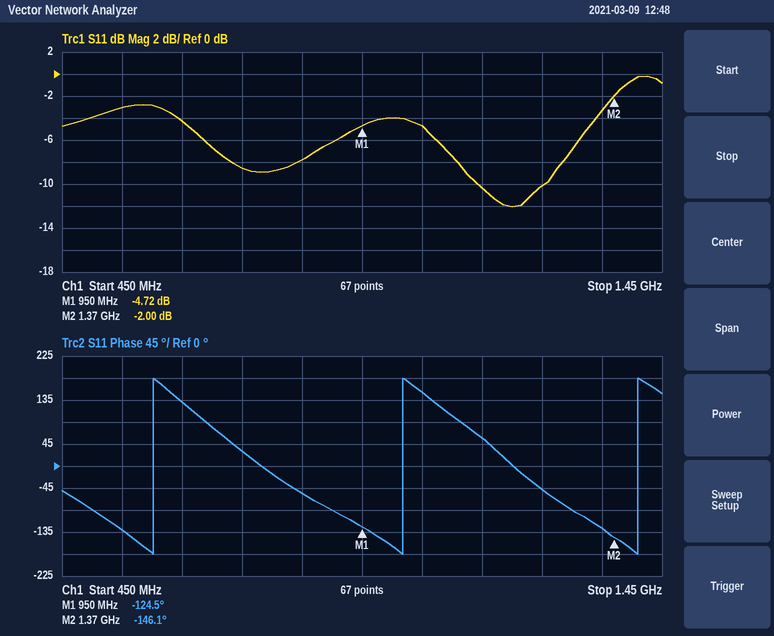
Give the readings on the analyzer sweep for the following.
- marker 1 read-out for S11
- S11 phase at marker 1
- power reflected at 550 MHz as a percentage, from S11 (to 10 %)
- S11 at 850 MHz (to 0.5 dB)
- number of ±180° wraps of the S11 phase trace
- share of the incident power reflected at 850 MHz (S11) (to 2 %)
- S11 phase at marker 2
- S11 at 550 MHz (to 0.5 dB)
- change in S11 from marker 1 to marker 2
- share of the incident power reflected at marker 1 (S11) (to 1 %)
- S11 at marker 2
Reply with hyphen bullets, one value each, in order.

- -4.72 dB
- -124.5°
- 50 %
- -8.0 dB
- 3
- 16 %
- -146.1°
- -3.0 dB
- 2.72 dB
- 34 %
- -2.00 dB
